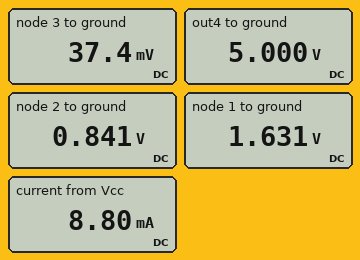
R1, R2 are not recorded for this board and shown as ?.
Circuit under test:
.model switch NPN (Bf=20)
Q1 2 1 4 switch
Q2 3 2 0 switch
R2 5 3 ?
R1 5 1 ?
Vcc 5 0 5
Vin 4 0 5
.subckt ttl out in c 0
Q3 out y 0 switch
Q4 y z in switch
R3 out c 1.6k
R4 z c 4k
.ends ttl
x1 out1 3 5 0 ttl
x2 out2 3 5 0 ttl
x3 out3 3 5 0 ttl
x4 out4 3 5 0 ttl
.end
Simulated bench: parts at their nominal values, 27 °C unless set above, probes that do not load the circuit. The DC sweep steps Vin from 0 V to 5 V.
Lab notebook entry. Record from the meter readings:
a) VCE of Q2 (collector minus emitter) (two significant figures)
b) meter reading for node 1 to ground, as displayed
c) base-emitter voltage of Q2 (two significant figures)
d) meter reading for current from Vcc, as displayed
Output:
37 mV
1.631 V
840 mV
8.80 mA
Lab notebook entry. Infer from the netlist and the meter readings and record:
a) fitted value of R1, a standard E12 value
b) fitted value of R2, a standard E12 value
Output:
1.8 kΩ
1.8 kΩ
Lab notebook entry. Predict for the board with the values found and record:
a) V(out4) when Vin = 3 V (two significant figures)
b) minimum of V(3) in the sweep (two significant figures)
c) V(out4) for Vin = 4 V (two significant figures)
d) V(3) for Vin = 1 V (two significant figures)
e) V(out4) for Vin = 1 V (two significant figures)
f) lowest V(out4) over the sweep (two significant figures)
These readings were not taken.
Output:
5.0 V
37 mV
5.0 V
37 mV
5.0 V
40 mV
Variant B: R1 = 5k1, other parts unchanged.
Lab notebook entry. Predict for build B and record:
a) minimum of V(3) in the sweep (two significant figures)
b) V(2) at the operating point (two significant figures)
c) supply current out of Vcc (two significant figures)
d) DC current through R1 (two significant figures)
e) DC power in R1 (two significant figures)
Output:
59 mV
830 mV
7.6 mA
670 µA
2.3 mW
